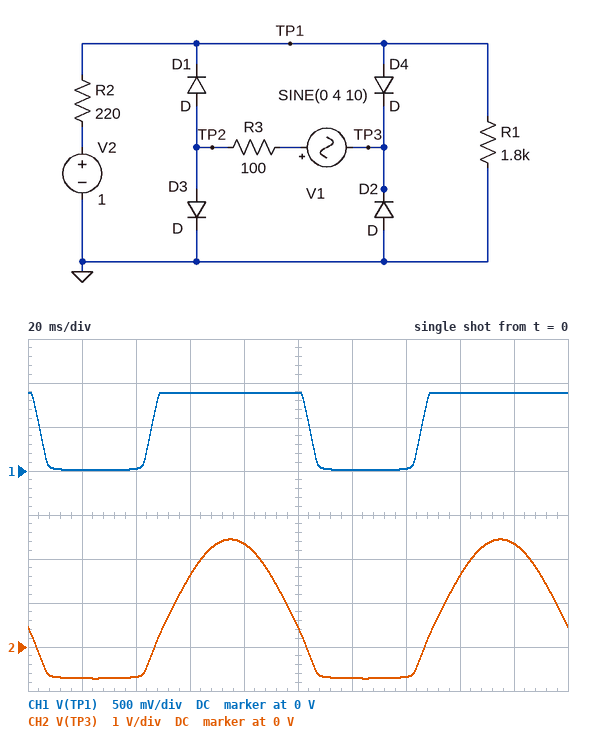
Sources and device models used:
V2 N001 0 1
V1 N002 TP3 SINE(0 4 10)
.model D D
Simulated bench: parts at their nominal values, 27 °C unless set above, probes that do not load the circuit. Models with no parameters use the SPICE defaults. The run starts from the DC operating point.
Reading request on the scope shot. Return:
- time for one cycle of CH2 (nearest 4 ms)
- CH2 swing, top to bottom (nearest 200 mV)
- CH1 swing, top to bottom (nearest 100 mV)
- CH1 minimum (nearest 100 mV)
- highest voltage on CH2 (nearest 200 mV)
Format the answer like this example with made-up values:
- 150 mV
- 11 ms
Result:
- 100 ms
- 3.2 V
- 900 mV
- 0 V
- 2.4 V
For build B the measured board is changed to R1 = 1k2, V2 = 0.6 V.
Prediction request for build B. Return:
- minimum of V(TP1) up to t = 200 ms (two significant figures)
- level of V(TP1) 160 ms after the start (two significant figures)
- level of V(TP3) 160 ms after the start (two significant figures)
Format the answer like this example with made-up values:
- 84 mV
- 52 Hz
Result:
- 5.5 mV
- 510 mV
- 1.4 V
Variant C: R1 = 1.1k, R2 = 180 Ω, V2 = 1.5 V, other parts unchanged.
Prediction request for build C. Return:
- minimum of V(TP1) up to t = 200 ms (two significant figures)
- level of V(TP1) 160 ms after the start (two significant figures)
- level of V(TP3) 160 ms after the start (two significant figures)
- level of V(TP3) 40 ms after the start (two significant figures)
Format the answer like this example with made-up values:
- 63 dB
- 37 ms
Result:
- 17 mV
- 1.3 V
- 1.8 V
- -650 mV
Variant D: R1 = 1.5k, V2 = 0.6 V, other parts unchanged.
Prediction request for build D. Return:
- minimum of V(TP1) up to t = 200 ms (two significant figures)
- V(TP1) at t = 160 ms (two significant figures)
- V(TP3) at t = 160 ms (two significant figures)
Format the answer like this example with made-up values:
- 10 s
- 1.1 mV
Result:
- 5.5 mV
- 520 mV
- 1.4 V
